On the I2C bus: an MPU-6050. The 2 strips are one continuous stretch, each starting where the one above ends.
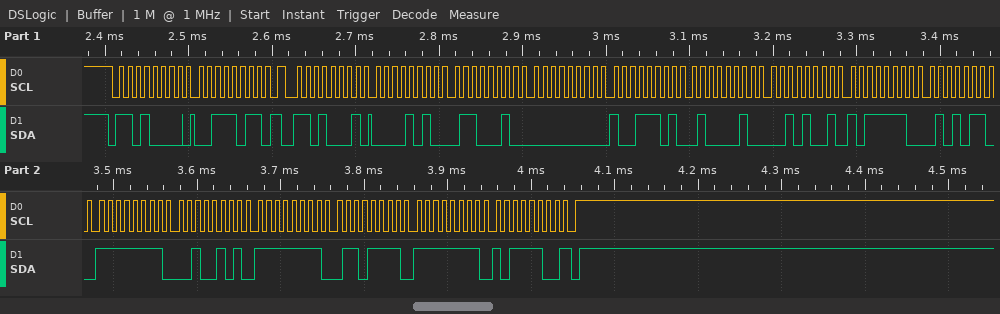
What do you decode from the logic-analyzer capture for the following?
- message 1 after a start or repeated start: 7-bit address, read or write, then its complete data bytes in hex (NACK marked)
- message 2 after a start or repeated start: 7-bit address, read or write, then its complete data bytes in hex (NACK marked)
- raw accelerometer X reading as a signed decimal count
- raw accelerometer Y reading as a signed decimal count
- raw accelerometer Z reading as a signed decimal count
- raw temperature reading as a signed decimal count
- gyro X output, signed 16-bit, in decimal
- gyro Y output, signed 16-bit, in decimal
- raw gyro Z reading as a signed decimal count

0x68 write: 3B
0x68 read: 0A 62 00 9D 42 29 BE 56 FF 25 FF 6F FF BC NACK
2658
157
16937
-16810
-219
-145
-68
